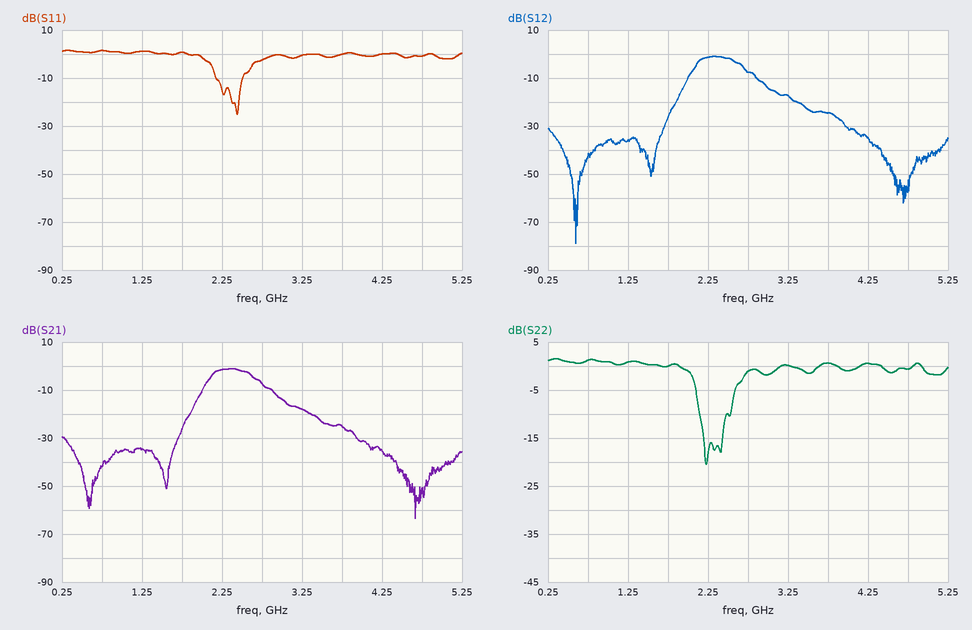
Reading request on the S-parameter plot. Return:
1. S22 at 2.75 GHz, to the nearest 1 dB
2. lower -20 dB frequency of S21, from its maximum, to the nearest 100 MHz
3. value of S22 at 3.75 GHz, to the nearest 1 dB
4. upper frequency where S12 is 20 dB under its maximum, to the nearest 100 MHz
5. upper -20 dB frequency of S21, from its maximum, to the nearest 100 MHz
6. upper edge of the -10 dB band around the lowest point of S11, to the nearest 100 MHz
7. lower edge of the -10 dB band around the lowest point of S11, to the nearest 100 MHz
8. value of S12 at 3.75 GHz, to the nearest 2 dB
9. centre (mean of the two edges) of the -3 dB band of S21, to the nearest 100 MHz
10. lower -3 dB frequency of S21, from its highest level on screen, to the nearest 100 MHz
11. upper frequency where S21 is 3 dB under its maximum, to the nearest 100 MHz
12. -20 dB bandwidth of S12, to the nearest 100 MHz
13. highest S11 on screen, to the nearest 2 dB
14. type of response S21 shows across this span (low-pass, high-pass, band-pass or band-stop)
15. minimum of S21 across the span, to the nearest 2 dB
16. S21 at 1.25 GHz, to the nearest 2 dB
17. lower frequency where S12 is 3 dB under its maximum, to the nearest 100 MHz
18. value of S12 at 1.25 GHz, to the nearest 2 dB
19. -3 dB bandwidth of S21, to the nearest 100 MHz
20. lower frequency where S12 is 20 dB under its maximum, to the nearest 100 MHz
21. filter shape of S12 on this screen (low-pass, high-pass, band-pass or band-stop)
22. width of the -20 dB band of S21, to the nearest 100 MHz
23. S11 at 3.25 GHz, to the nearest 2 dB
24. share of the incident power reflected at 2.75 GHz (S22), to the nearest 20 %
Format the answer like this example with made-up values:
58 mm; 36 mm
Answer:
-1 dB; 1.8 GHz; 1 dB; 3.4 GHz; 3.4 GHz; 2.5 GHz; 2.2 GHz; -24 dB; 2.4 GHz; 2.1 GHz; 2.6 GHz; 1.6 GHz; 2 dB; band-pass; -64 dB; -34 dB; 2.1 GHz; -36 dB; 500 MHz; 1.8 GHz; band-pass; 1.6 GHz; 0 dB; 80 %
